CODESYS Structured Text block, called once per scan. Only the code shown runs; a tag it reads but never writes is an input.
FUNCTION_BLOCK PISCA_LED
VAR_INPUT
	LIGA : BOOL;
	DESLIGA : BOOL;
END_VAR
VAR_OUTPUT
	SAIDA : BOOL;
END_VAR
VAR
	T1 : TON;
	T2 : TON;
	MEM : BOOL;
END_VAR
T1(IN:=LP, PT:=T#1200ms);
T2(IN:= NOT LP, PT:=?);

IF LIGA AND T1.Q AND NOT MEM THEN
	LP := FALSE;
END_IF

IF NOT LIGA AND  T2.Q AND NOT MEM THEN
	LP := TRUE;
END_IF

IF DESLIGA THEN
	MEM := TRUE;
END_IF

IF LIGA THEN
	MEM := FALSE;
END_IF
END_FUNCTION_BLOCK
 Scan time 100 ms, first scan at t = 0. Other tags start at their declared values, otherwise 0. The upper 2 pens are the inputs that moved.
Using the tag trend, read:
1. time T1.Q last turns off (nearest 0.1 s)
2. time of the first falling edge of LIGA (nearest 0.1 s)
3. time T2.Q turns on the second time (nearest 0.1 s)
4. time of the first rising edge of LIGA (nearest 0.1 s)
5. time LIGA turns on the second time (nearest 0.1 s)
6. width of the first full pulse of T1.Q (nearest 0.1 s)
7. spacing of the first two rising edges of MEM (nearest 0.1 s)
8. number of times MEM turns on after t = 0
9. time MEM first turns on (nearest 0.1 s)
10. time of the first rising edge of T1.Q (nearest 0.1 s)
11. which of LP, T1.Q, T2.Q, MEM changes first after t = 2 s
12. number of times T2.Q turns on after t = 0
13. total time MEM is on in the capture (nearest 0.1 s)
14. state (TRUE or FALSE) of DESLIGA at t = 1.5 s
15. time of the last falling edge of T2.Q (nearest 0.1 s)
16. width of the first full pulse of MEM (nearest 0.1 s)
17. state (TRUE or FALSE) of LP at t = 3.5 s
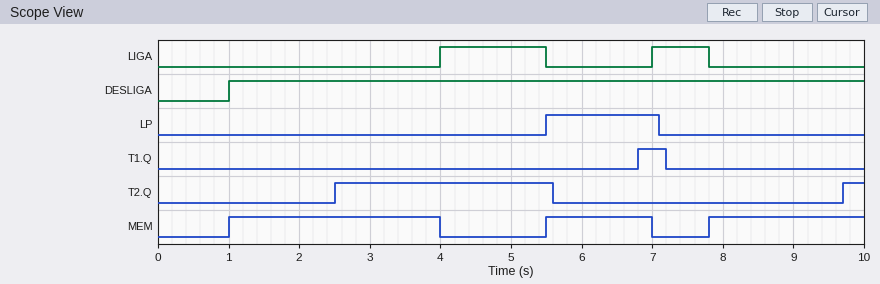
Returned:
7.2 s
5.5 s
9.7 s
4.0 s
7.0 s
0.4 s
4.5 s
3
1.0 s
6.8 s
T2.Q
2
6.7 s
TRUE
5.6 s
3.0 s
FALSE
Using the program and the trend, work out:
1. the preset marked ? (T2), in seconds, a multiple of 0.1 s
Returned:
2.5 s
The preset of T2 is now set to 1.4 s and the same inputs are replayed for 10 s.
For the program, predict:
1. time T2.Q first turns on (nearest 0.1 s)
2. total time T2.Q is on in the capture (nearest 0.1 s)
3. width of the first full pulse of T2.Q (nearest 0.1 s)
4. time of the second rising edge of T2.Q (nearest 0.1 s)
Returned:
1.4 s
5.6 s
4.2 s
8.6 s
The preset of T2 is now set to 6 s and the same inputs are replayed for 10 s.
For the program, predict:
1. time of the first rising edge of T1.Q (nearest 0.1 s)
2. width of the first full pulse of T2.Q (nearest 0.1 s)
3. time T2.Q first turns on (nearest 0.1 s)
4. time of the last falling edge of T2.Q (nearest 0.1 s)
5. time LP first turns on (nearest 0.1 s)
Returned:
9.1 s
1.9 s
6.0 s
7.9 s
7.8 s
